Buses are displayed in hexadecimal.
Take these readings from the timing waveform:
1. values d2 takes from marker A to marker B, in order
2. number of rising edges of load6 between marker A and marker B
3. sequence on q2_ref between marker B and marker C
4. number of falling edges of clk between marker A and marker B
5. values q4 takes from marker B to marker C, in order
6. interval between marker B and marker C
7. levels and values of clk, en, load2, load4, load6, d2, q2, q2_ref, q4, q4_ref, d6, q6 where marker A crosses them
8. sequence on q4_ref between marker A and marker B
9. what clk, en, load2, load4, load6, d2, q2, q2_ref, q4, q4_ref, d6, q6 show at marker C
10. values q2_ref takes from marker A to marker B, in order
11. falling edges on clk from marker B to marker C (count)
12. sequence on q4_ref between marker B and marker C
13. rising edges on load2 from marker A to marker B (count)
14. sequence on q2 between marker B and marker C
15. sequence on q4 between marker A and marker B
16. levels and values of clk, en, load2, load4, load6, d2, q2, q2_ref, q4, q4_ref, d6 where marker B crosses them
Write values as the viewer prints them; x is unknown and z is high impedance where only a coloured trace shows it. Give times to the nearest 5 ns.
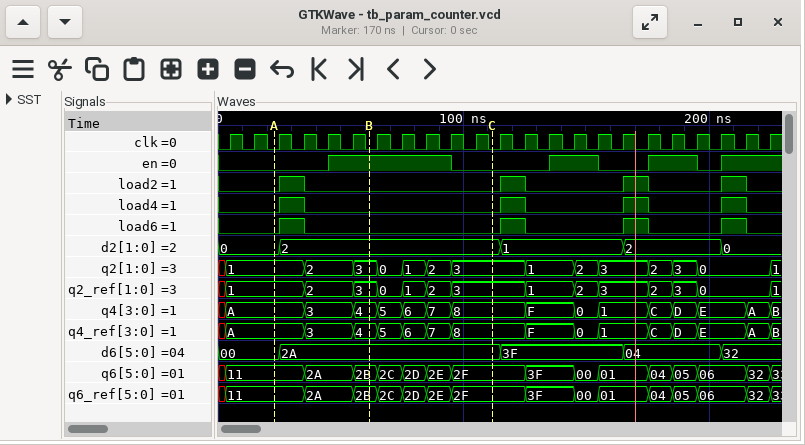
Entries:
0, 2
1
3, 0, 1, 2, 3
4
4, 5, 6, 7, 8
50 ns
clk=0, en=0, load2=0, load4=0, load6=0, d2=0, q2=1, q2_ref=1, q4=A, q4_ref=A, d6=00, q6=11
A, 3, 4
clk=0, en=0, load2=0, load4=0, load6=0, d2=2, q2=3, q2_ref=3, q4=8, q4_ref=8, d6=2A, q6=2F
1, 2, 3
5
4, 5, 6, 7, 8
1
3, 0, 1, 2, 3
A, 3, 4
clk=0, en=1, load2=0, load4=0, load6=0, d2=2, q2=3, q2_ref=3, q4=4, q4_ref=4, d6=2A
